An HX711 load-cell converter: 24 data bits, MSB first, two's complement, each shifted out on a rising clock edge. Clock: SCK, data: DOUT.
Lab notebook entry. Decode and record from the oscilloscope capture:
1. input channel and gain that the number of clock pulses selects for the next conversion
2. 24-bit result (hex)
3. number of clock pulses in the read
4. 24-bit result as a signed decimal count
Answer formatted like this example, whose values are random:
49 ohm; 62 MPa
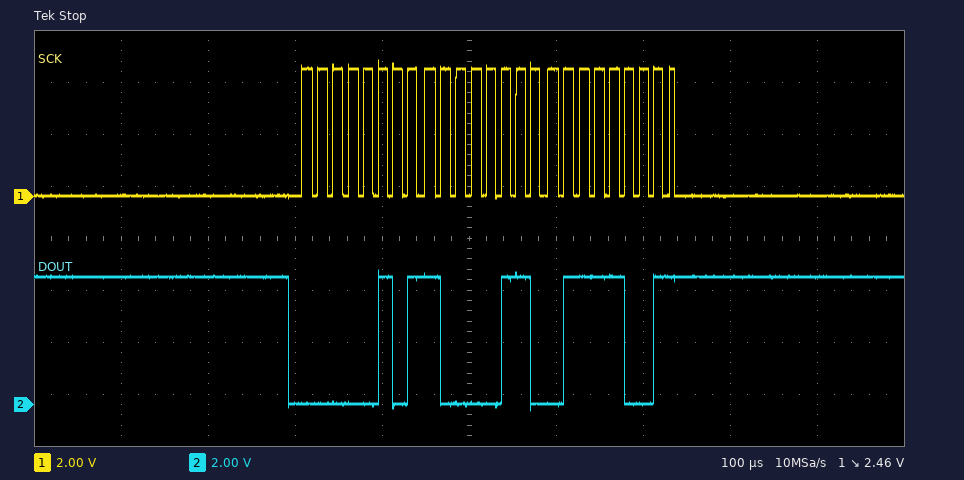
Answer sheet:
channel A, gain 128; 0x058679; 25; 362105
